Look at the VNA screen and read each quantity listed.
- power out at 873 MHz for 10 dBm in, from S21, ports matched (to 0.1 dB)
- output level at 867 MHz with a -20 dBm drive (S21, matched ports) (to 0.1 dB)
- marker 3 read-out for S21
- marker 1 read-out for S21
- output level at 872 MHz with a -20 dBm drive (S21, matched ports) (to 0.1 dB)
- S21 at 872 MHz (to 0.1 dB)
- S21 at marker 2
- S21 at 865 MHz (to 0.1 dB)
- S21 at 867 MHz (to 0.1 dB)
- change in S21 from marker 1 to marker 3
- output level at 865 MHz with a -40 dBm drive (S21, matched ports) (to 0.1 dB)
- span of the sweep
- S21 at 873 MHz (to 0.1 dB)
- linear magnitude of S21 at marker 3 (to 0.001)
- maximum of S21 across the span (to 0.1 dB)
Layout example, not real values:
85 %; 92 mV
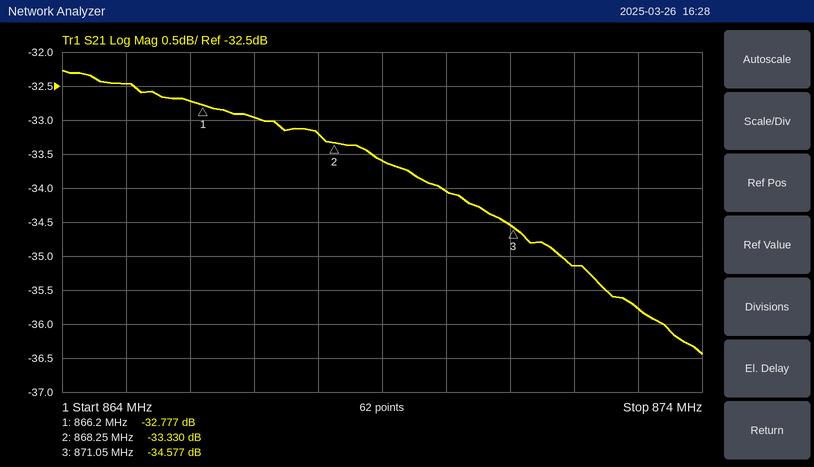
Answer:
-25.8 dBm; -53.0 dBm; -34.577 dB; -32.777 dB; -55.1 dBm; -35.1 dB; -33.330 dB; -32.5 dB; -33.0 dB; -1.800 dB; -72.5 dBm; 10 MHz; -35.8 dB; 0.019; -32.3 dB
